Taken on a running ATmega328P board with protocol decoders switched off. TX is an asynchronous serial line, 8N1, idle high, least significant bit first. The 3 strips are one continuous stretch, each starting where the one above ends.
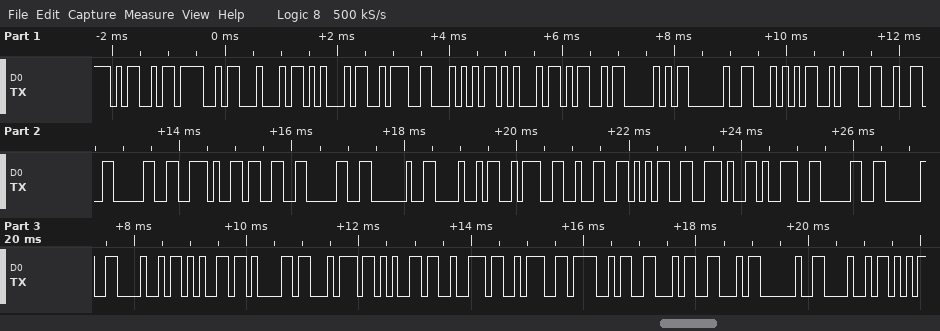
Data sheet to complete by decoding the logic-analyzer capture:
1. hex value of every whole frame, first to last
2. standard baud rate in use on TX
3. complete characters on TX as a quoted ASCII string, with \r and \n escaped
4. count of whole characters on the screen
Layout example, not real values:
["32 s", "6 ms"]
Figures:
["4D 4F 44 45 3A 54 45 4D 50 20 54 3A 32 30 2E 33 30 20 48 3A 32 35 2E 39 30 20 48 65 61 74 65 72 3A 4F 46 46 20 48", "9600 baud", "\"MODE:TEMP T:20.30 H:25.90 Heater:OFF H\"", "38"]
